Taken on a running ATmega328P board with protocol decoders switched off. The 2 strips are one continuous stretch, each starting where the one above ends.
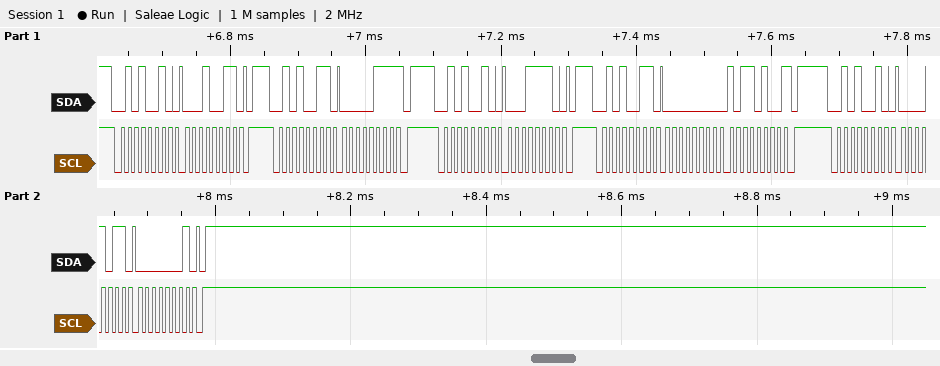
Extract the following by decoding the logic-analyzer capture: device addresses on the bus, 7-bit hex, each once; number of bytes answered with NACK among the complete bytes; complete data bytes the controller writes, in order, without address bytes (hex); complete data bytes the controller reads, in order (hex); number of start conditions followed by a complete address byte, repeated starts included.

0x29
2
13 1E 0B 01
07 00 B4
5
